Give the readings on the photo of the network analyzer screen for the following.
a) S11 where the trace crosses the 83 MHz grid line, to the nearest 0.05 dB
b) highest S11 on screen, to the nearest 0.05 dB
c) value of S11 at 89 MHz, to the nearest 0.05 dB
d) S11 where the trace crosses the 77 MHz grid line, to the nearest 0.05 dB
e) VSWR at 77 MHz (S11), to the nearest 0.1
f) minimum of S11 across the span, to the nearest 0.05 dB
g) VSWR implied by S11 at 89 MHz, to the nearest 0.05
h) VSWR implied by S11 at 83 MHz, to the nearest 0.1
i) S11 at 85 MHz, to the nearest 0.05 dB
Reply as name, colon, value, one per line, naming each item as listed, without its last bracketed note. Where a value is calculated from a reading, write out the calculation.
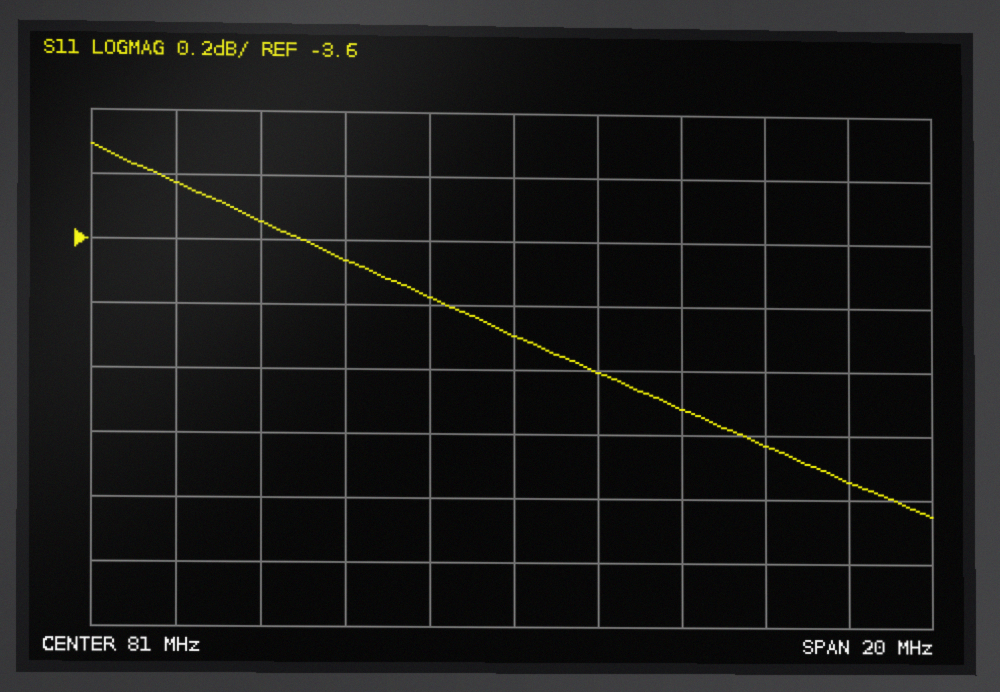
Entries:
S11 where the trace crosses the 83 MHz grid line, to the nearest 0.05 dB: -4.00 dB
highest S11 on screen, to the nearest 0.05 dB: -3.30 dB
value of S11 at 89 MHz, to the nearest 0.05 dB: -4.35 dB
S11 where the trace crosses the 77 MHz grid line, to the nearest 0.05 dB: -3.65 dB
VSWR at 77 MHz (S11), to the nearest 0.1: |Γ| = 10^(-3.65/20) = 0.6569; VSWR = (1 + 0.6569)/(1 − 0.6569) ≈ 4.8
minimum of S11 across the span, to the nearest 0.05 dB: -4.45 dB
VSWR implied by S11 at 89 MHz, to the nearest 0.05: |Γ| = 10^(-4.35/20) = 0.6060; VSWR = (1 + 0.6060)/(1 − 0.6060) ≈ 4.08, so 4.10 to the nearest 0.05
VSWR implied by S11 at 83 MHz, to the nearest 0.1: |Γ| = 10^(-4/20) = 0.6310; VSWR = (1 + 0.6310)/(1 − 0.6310) ≈ 4.4
S11 at 85 MHz, to the nearest 0.05 dB: -4.10 dB
